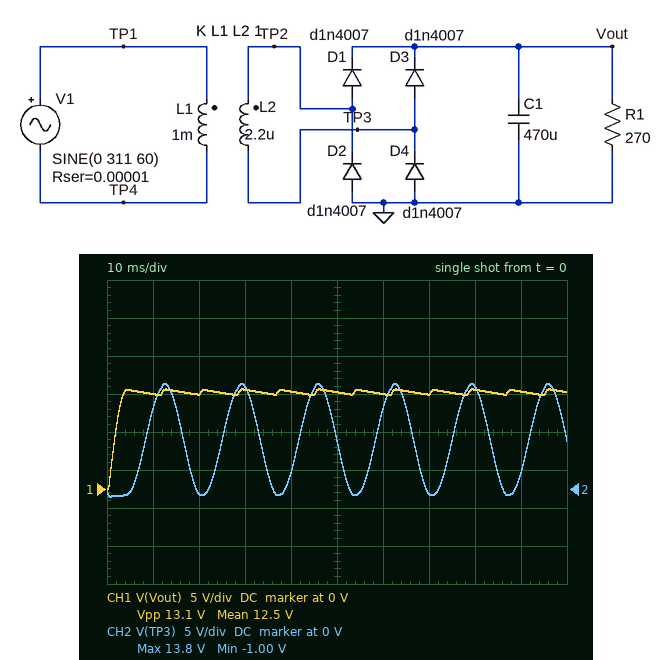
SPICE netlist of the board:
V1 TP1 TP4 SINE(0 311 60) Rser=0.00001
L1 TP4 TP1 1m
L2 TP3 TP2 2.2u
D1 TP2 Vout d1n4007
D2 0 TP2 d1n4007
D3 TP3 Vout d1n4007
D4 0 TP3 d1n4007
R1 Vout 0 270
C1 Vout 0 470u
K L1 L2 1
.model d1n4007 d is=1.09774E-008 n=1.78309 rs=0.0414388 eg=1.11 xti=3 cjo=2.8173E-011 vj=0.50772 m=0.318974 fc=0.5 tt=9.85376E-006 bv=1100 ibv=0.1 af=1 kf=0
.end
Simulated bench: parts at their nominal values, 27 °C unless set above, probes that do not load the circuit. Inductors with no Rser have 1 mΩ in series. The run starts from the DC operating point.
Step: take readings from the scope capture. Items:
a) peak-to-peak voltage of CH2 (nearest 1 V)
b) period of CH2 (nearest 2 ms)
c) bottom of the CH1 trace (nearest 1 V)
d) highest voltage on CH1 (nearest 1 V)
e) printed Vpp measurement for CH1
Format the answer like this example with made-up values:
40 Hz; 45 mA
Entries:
15 V; 16 ms; 0 V; 13 V; 13.1 V
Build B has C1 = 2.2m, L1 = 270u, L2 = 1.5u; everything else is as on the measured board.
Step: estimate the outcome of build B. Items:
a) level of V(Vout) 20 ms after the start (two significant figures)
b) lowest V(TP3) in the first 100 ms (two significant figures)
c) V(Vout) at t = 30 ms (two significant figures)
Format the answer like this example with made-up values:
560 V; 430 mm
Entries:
21 V; -1.7 V; 22 V
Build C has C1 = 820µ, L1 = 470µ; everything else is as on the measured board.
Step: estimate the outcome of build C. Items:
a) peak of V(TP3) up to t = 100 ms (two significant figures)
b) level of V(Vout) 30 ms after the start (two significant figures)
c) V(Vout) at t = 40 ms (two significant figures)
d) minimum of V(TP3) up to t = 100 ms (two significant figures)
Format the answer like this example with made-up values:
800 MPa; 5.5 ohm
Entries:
21 V; 20 V; 19 V; -1.2 V
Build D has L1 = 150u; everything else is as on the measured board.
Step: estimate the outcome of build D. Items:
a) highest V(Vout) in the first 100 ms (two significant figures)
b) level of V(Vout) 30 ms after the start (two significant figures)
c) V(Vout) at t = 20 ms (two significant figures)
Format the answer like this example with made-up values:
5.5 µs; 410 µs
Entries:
37 V; 36 V; 35 V
